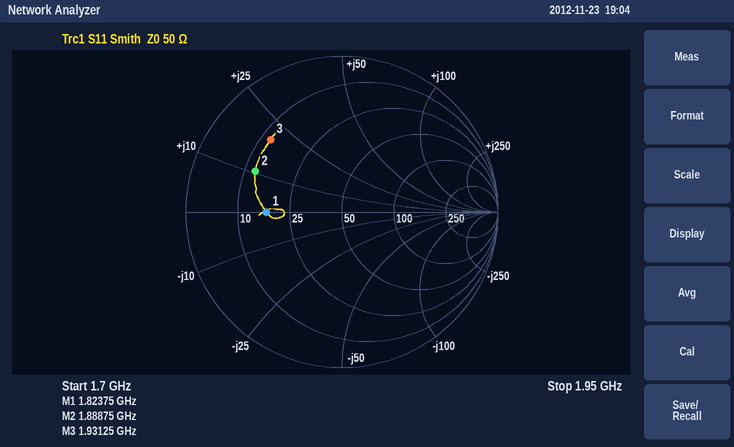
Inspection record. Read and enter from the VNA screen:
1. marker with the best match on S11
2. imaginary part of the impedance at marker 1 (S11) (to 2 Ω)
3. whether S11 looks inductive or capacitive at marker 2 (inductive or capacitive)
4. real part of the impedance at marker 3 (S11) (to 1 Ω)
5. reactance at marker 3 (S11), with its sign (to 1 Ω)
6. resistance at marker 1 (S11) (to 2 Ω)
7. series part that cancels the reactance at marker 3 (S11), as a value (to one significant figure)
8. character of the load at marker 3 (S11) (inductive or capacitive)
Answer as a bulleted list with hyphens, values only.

- marker 1
- 0 Ω
- inductive
- 12 Ω
- +20 Ω
- 18 Ω
- 4 pF
- inductive
